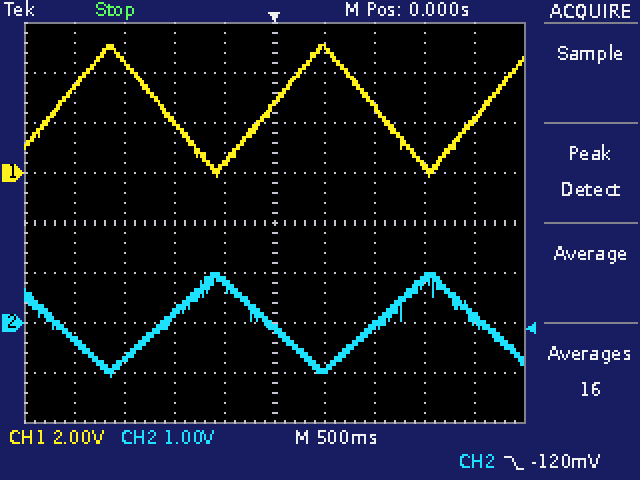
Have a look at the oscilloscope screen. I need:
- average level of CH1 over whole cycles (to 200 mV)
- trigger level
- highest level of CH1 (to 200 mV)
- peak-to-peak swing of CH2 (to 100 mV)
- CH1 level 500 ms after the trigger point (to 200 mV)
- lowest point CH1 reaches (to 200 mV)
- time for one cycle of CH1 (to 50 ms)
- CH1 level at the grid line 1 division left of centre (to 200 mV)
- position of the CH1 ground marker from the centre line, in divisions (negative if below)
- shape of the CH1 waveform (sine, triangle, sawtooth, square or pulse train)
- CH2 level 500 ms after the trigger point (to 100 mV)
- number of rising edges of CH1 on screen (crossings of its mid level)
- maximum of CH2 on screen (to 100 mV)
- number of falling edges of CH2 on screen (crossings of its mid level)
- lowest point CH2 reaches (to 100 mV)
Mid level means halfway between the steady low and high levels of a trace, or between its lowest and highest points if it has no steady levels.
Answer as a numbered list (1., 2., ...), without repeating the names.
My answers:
1. 2.6 V
2. -120 mV
3. 5.2 V
4. 2.1 V
5. 5.0 V
6. -200 mV
7. 2.15 s
8. 400 mV
9. +1.0 div
10. triangle
11. -900 mV
12. 3
13. 1.0 V
14. 3
15. -1.1 V
